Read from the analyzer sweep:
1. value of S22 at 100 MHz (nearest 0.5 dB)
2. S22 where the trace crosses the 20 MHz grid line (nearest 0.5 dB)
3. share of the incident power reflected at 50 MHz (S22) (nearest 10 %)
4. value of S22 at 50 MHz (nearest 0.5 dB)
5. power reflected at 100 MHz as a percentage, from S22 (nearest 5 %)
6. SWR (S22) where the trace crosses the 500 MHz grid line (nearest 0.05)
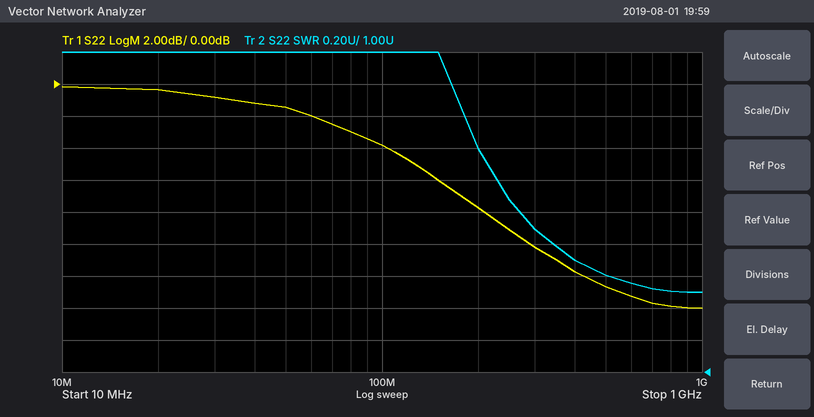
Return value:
-4.0 dB
-0.5 dB
70 %
-1.5 dB
40 %
1.60
